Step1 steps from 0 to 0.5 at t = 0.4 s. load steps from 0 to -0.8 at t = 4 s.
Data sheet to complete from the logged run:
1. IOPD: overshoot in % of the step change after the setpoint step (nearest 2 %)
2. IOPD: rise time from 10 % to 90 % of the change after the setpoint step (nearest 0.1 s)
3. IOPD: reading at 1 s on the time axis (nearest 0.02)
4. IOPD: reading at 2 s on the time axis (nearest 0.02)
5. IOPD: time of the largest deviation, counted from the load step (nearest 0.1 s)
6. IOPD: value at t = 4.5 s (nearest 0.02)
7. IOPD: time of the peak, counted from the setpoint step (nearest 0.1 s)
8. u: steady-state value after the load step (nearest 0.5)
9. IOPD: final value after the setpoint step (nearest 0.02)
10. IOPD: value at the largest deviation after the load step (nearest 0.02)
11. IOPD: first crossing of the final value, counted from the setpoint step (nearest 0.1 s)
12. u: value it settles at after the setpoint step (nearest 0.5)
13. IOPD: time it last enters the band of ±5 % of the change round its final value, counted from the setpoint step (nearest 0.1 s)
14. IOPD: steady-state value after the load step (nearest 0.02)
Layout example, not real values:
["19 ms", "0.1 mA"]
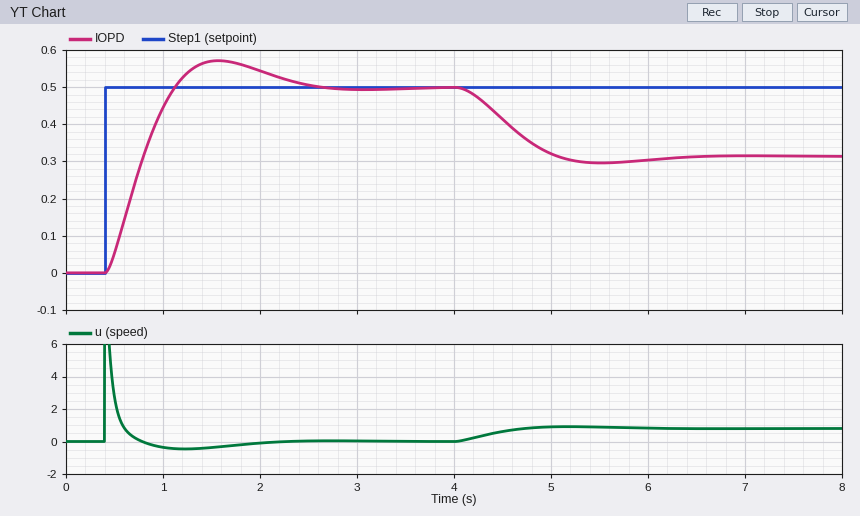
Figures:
["14 %", "0.5 s", "0.44", "0.54", "1.5 s", "0.42", "1.2 s", "1.0", "0.50", "0.30", "0.7 s", "0.0", "1.8 s", "0.32"]
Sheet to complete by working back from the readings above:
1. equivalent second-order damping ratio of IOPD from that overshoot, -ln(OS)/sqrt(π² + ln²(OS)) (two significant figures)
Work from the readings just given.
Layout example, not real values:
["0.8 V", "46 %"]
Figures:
["0.53"]
